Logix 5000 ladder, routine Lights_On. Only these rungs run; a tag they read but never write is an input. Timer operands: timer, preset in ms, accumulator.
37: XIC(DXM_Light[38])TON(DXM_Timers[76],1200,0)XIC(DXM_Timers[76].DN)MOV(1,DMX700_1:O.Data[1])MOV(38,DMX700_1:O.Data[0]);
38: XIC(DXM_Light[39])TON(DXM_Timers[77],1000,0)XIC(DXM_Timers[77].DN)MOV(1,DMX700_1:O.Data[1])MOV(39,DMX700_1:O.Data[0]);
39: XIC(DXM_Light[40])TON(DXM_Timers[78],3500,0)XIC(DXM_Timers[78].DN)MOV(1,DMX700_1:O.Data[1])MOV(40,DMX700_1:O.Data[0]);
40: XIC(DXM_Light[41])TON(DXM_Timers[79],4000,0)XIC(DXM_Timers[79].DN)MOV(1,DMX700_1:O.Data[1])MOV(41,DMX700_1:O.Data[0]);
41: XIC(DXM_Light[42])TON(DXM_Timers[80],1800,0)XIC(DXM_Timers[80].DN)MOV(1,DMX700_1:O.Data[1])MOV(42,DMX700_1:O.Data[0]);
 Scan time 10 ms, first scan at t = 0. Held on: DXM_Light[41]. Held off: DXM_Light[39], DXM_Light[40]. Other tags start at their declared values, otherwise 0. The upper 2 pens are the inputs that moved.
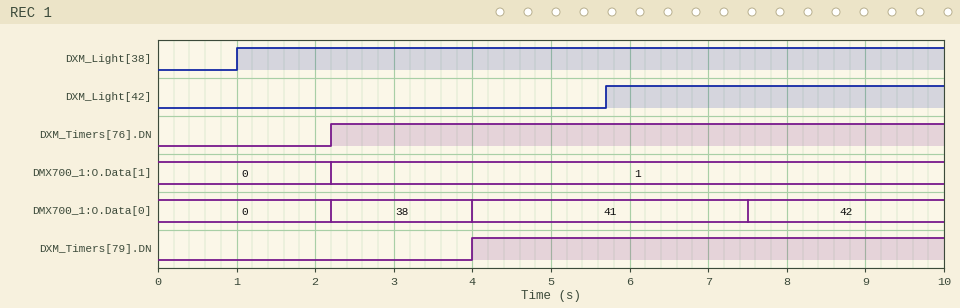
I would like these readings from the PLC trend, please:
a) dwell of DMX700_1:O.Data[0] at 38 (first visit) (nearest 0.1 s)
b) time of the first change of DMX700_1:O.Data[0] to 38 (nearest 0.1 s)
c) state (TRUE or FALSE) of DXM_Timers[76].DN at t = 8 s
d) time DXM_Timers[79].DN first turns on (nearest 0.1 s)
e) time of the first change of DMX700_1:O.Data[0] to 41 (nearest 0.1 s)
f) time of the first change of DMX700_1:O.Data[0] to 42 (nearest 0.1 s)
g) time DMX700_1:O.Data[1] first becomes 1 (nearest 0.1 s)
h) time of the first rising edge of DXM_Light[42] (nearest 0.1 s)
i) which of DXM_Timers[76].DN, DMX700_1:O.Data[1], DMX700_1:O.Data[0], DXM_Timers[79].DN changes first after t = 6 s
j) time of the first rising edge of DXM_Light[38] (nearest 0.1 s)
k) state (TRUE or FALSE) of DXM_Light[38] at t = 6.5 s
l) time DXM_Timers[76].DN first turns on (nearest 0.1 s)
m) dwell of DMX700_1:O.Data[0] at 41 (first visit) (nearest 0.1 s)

1.8 s
2.2 s
TRUE
4.0 s
4.0 s
7.5 s
2.2 s
5.7 s
DMX700_1:O.Data[0]
1.0 s
TRUE
2.2 s
3.5 s
